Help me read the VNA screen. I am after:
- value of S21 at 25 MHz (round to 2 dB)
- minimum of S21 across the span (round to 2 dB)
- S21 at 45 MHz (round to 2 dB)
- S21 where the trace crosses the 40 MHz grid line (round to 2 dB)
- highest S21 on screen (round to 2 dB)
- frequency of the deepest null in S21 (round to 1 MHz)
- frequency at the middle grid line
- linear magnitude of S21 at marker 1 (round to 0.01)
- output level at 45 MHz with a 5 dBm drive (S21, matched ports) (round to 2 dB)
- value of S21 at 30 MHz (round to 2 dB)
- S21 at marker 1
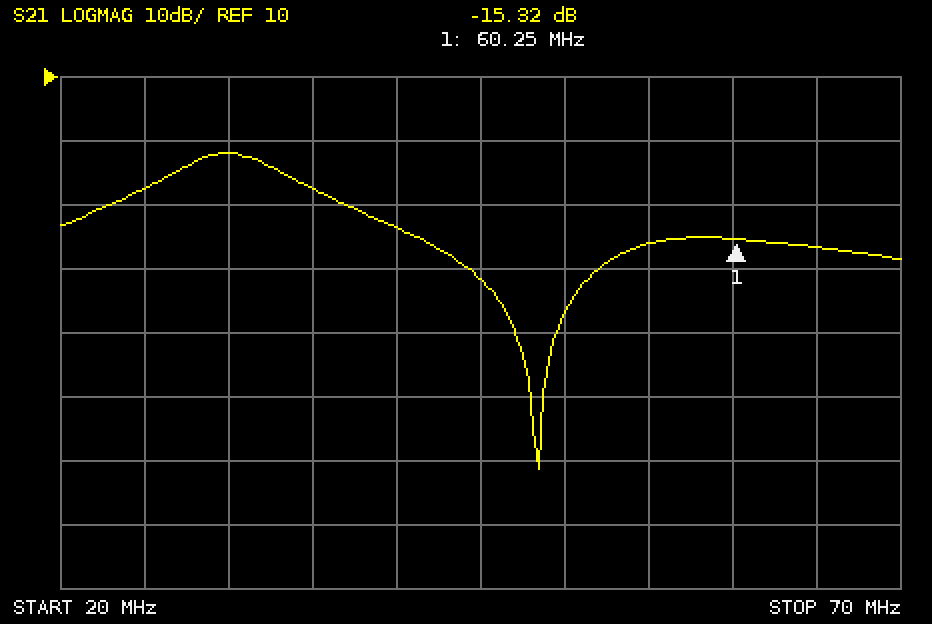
-8 dB
-52 dB
-22 dB
-14 dB
-2 dB
48 MHz
45 MHz
0.17
-16 dBm
-2 dB
-15.32 dB
